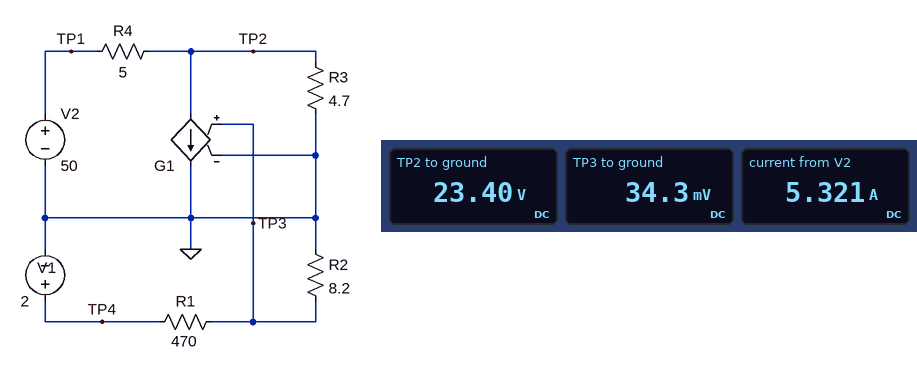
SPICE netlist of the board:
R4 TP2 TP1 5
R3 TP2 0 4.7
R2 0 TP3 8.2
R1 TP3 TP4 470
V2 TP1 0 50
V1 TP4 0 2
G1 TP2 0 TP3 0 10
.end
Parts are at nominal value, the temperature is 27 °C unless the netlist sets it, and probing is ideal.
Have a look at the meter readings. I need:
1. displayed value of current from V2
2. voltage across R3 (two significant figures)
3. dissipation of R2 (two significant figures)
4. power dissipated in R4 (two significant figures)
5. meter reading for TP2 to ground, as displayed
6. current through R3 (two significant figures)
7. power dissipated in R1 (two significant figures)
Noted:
5.321 A
23 V
140 µW
140 W
23.40 V
5.0 A
8.2 mW
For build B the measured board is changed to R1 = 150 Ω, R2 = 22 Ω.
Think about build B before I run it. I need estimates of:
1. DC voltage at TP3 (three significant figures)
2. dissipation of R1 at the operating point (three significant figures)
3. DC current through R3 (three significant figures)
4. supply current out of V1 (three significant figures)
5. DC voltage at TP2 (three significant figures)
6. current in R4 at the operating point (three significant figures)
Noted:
256 mV
20.3 mW
3.84 A
11.6 mA
18.0 V
6.39 A
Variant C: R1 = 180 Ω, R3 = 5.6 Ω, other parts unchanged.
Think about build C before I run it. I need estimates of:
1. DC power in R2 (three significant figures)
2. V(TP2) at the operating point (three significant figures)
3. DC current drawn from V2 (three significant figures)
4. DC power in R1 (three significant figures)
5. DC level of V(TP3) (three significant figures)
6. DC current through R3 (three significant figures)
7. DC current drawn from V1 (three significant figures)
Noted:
926 µW
24.1 V
5.18 A
20.3 mW
87.1 mV
4.31 A
10.6 mA
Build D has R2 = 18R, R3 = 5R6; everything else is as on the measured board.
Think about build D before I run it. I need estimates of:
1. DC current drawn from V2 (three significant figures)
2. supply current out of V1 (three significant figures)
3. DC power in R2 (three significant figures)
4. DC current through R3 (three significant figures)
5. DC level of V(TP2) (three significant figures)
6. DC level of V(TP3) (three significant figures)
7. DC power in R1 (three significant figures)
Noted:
5.11 A
4.10 mA
302 µW
4.37 A
24.5 V
73.8 mV
7.89 mW
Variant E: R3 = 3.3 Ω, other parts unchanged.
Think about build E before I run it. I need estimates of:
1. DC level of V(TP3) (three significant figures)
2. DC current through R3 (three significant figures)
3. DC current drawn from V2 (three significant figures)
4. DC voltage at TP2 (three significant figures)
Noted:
34.3 mV
5.82 A
6.16 A
19.2 V
